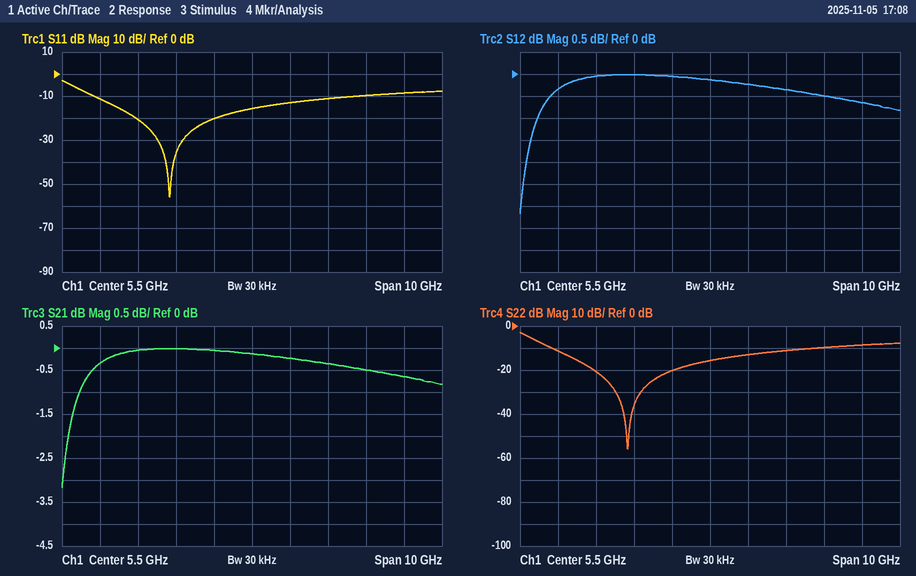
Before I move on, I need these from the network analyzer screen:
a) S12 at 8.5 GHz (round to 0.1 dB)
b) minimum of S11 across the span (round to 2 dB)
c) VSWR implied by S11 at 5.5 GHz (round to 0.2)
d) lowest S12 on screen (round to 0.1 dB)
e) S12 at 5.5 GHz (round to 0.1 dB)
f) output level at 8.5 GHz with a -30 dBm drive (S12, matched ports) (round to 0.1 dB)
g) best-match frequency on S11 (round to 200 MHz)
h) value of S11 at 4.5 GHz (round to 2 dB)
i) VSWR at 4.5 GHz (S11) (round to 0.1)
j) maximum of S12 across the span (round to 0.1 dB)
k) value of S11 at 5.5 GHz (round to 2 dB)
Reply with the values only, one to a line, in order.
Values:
-0.5 dB
-56 dB
1.4
-3.2 dB
-0.1 dB
-30.5 dBm
3.4 GHz
-20 dB
1.2
0.0 dB
-16 dB
